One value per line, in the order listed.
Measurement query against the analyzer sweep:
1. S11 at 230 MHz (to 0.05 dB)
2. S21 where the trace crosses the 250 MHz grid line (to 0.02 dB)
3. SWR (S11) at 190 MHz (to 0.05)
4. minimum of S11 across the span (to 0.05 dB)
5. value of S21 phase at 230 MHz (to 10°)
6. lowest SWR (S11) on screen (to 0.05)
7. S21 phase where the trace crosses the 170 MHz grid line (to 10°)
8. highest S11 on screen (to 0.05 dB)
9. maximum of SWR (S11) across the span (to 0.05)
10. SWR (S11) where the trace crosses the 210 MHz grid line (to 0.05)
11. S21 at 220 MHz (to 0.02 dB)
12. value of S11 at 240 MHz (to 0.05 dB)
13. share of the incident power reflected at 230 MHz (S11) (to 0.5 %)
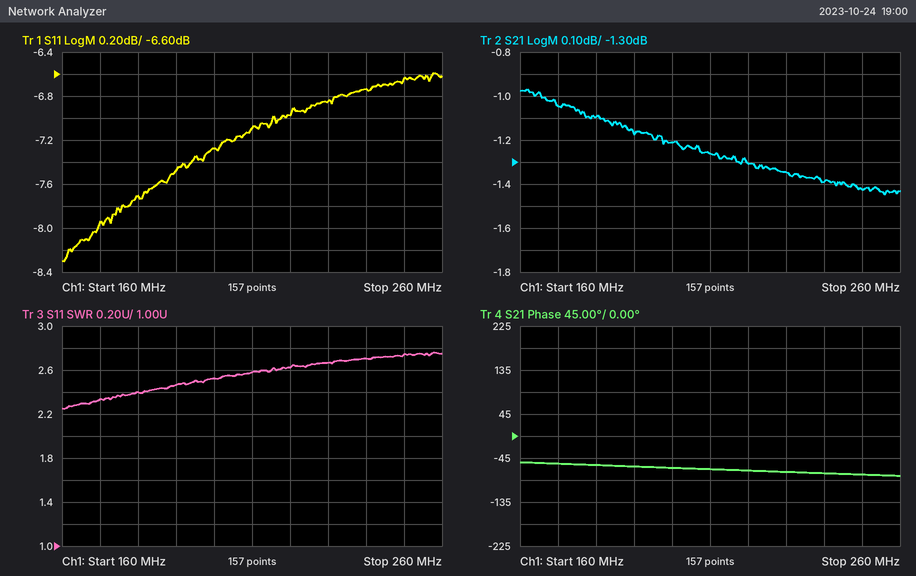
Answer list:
-6.85 dB
-1.42 dB
2.45
-8.30 dB
-70°
2.25
-60°
-6.60 dB
2.75
2.60
-1.30 dB
-6.75 dB
20.5 %
